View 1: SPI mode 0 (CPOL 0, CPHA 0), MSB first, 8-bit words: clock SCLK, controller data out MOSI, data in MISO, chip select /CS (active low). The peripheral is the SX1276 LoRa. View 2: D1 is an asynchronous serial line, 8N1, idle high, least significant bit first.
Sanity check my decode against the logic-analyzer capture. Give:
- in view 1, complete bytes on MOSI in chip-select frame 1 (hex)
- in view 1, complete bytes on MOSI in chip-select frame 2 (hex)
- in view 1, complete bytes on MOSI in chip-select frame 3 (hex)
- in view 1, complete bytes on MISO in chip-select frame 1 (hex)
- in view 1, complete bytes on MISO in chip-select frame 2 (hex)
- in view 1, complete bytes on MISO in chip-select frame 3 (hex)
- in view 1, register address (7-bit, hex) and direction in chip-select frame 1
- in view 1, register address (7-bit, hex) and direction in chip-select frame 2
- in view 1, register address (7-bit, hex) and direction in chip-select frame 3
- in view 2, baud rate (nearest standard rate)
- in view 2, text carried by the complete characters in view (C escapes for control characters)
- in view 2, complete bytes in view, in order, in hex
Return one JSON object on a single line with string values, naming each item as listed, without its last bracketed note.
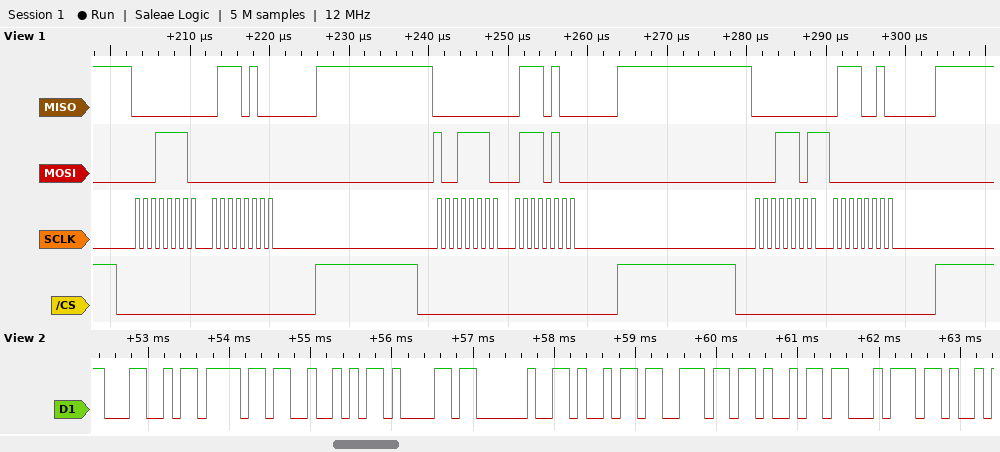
{"in view 1, complete bytes on MOSI in chip-select frame 1": "1E 00", "in view 1, complete bytes on MOSI in chip-select frame 2": "9E 74", "in view 1, complete bytes on MOSI in chip-select frame 3": "1D 00", "in view 1, complete bytes on MISO in chip-select frame 1": "00 74", "in view 1, complete bytes on MISO in chip-select frame 2": "00 74", "in view 1, complete bytes on MISO in chip-select frame 3": "00 72", "in view 1, register address (7-bit, hex) and direction in chip-select frame 1": "0x1E read", "in view 1, register address (7-bit, hex) and direction in chip-select frame 2": "0x1E write", "in view 1, register address (7-bit, hex) and direction in chip-select frame 3": "0x1D read", "in view 2, baud rate": "9600 baud", "in view 2, text carried by the complete characters in view": "\"LoRa init\"", "in view 2, complete bytes in view, in order, in hex": "4C 6F 52 61 20 69 6E 69 74"}
